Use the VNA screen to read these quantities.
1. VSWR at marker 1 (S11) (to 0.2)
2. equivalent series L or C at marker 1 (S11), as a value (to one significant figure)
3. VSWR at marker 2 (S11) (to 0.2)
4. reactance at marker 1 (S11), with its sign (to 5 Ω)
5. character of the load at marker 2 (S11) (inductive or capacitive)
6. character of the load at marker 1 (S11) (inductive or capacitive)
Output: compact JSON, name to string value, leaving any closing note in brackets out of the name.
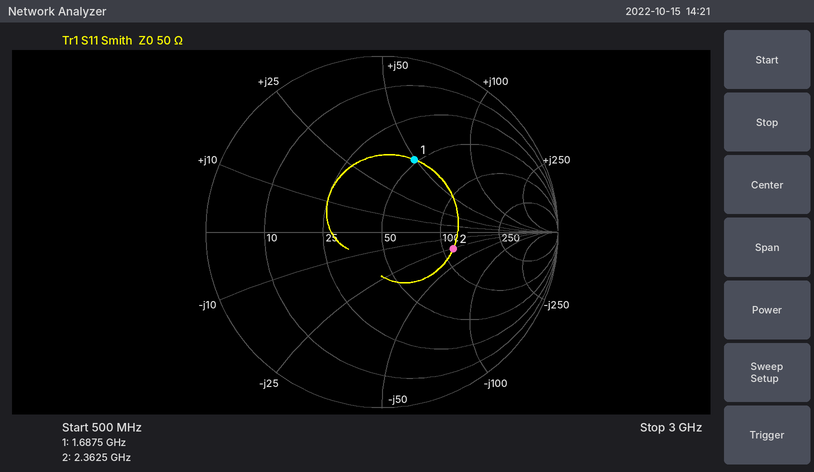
{"VSWR at marker 1 (S11)": "2.6", "equivalent series L or C at marker 1 (S11), as a value": "5 nH", "VSWR at marker 2 (S11)": "2.4", "reactance at marker 1 (S11), with its sign": "+50 Ω", "character of the load at marker 2 (S11)": "capacitive", "character of the load at marker 1 (S11)": "inductive"}
